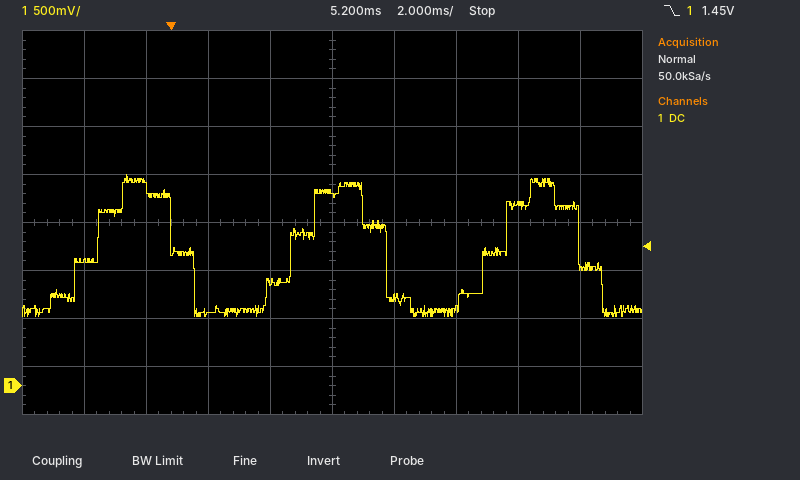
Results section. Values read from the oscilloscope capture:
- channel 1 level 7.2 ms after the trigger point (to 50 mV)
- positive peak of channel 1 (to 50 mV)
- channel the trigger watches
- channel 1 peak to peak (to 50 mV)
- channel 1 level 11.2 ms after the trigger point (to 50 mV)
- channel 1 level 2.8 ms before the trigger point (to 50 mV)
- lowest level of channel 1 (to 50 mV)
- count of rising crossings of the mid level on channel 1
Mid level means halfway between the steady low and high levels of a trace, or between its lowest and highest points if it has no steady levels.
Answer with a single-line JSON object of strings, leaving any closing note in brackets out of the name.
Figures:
{"channel 1 level 7.2 ms after the trigger point": "900 mV", "positive peak of channel 1": "2.20 V", "channel the trigger watches": "channel 1", "channel 1 peak to peak": "1.50 V", "channel 1 level 11.2 ms after the trigger point": "1.90 V", "channel 1 level 2.8 ms before the trigger point": "1.30 V", "lowest level of channel 1": "700 mV", "count of rising crossings of the mid level on channel 1": "3"}
